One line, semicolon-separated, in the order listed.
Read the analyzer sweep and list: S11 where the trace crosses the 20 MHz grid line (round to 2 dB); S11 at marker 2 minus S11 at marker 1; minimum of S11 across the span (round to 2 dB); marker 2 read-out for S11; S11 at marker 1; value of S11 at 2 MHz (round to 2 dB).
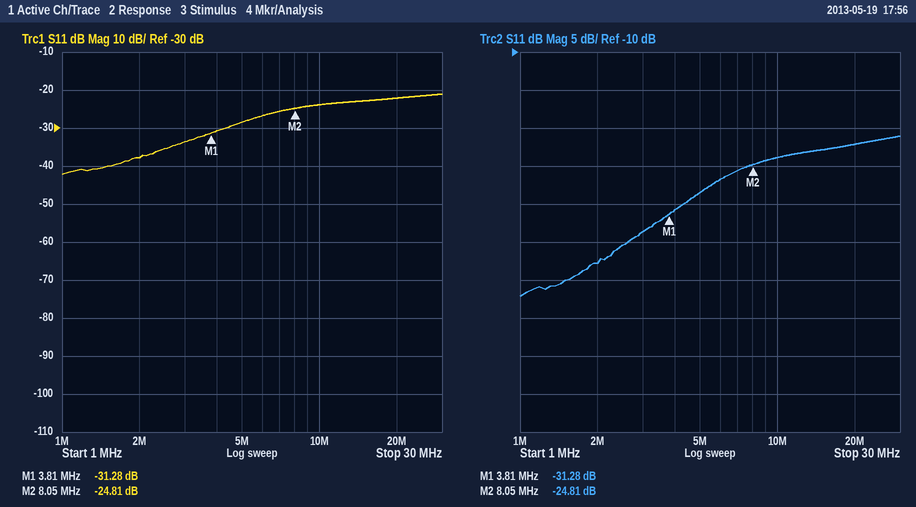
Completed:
-22 dB; 6.47 dB; -42 dB; -24.81 dB; -31.28 dB; -38 dB
